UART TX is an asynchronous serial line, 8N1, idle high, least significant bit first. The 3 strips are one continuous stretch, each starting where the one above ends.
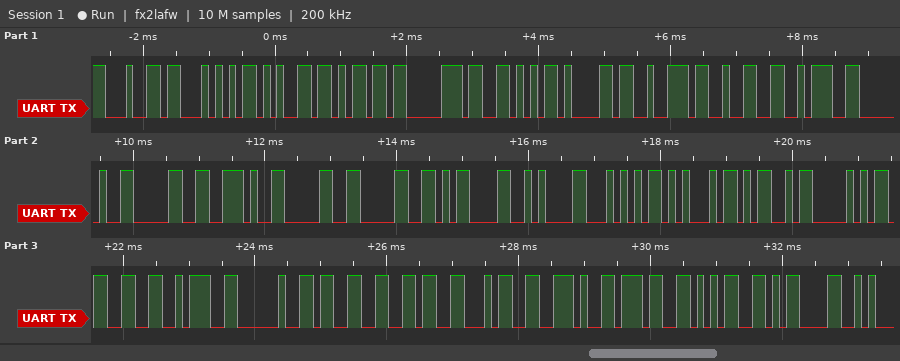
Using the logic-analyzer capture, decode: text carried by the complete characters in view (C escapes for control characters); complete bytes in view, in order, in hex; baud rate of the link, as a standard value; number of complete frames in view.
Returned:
"dTempVar2: 0.00\r\nTEMP3: 364.75\r"
0x64 0x54 0x65 0x6D 0x70 0x56 0x61 0x72 0x32 0x3A 0x20 0x30 0x2E 0x30 0x30 0x0D 0x0A 0x54 0x45 0x4D 0x50 0x33 0x3A 0x20 0x33 0x36 0x34 0x2E 0x37 0x35 0x0D
9600 baud
31
